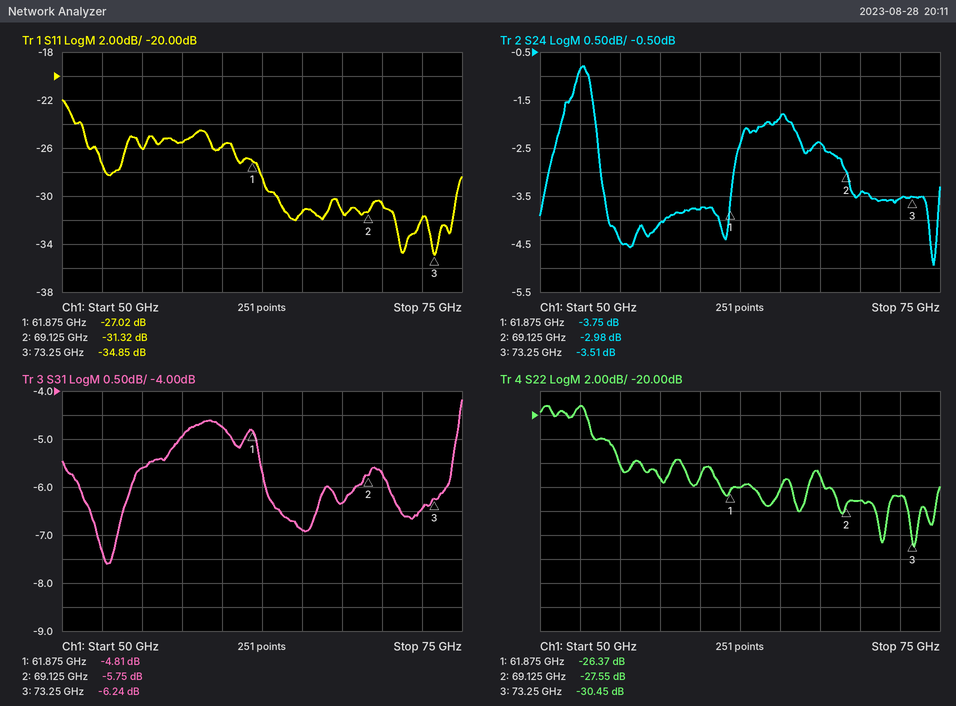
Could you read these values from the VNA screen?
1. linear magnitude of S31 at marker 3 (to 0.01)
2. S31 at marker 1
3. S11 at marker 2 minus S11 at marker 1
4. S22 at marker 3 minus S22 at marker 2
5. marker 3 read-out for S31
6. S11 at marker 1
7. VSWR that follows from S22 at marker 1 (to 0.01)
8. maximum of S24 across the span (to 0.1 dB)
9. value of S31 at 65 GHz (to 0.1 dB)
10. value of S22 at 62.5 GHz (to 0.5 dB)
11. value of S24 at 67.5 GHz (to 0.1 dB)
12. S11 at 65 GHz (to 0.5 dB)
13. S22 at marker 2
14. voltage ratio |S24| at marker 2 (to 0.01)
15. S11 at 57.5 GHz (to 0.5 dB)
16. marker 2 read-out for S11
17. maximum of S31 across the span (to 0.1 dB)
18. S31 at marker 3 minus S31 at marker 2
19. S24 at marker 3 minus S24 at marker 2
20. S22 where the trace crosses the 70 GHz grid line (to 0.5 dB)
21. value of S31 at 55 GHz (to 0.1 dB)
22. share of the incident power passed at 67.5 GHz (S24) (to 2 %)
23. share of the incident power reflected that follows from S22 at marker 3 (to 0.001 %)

0.49
-4.81 dB
-4.30 dB
-2.90 dB
-6.24 dB
-27.02 dB
1.10
-0.8 dB
-6.9 dB
-26.0 dB
-2.4 dB
-31.5 dB
-27.55 dB
0.71
-25.5 dB
-31.32 dB
-4.2 dB
-0.49 dB
-0.53 dB
-27.0 dB
-5.6 dB
58 %
0.090 %
